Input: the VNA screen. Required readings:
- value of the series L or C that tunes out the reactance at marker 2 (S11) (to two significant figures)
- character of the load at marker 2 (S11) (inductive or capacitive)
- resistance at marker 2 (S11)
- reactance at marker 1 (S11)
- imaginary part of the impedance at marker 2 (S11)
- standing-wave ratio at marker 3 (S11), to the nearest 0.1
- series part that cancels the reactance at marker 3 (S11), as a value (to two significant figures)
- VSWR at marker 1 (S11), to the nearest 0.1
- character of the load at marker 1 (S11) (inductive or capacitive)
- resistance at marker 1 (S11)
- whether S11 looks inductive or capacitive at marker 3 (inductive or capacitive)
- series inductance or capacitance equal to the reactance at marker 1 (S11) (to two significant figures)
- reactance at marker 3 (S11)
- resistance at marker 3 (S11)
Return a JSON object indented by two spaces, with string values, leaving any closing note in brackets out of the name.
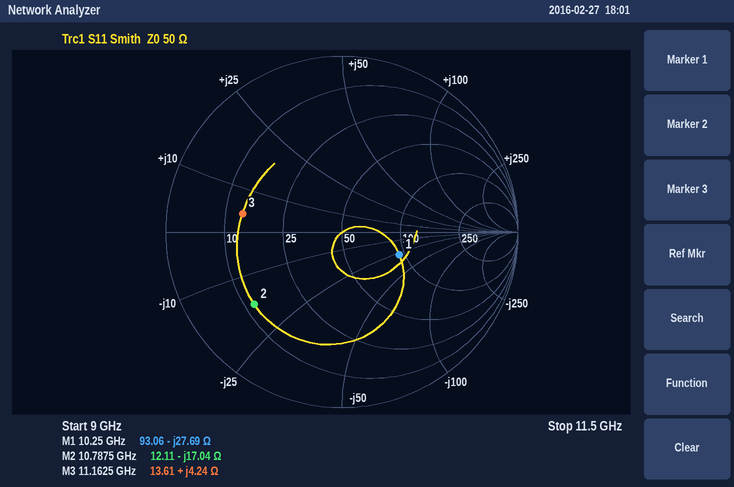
{
  "value of the series L or C that tunes out the reactance at marker 2 (S11)": "250 pH",
  "character of the load at marker 2 (S11)": "capacitive",
  "resistance at marker 2": "12.11 Ω",
  "reactance at marker 1": "-27.69 Ω",
  "imaginary part of the impedance at marker 2": "-17.04 Ω",
  "standing-wave ratio at marker 3 (S11), to the nearest 0.1": "3.7",
  "series part that cancels the reactance at marker 3 (S11), as a value": "3.4 pF",
  "VSWR at marker 1 (S11), to the nearest 0.1": "2.1",
  "character of the load at marker 1 (S11)": "capacitive",
  "resistance at marker 1": "93.06 Ω",
  "whether S11 looks inductive or capacitive at marker 3": "inductive",
  "series inductance or capacitance equal to the reactance at marker 1 (S11)": "560 fF",
  "reactance at marker 3": "+4.24 Ω",
  "resistance at marker 3": "13.61 Ω"
}
